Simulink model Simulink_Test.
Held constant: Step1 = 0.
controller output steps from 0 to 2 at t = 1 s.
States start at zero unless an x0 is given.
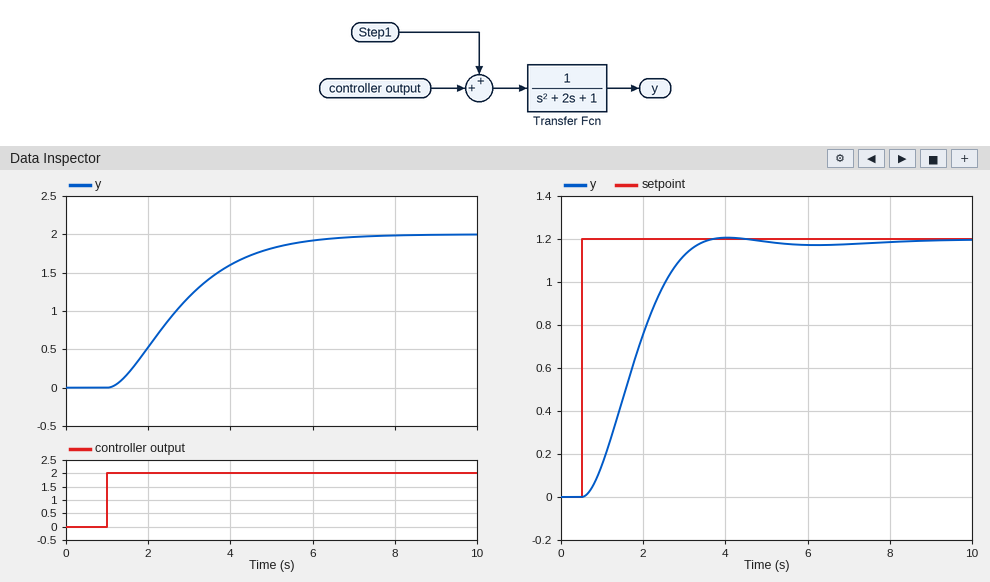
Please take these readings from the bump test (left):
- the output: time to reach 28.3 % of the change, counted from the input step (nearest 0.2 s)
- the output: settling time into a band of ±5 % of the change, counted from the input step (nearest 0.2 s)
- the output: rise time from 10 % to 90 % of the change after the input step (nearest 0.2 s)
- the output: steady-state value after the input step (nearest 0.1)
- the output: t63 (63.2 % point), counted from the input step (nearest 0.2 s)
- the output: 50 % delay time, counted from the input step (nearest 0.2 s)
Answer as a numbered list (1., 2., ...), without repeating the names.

1. 1.0 s
2. 4.8 s
3. 3.4 s
4. 2.0
5. 2.2 s
6. 1.6 s
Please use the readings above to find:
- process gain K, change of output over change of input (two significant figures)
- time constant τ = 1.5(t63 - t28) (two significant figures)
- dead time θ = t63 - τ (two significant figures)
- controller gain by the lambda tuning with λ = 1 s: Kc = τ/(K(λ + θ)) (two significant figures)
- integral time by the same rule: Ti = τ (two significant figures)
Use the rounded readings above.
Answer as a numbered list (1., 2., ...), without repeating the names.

1. 1.0
2. 1.8 s
3. 0.40 s
4. 1.3
5. 1.8 s
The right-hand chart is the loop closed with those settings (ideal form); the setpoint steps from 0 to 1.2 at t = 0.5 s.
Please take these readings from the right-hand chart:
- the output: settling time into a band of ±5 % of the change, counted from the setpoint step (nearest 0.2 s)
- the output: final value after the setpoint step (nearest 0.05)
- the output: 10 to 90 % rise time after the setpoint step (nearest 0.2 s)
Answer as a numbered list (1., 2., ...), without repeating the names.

1. 2.6 s
2. 1.20
3. 1.8 s
